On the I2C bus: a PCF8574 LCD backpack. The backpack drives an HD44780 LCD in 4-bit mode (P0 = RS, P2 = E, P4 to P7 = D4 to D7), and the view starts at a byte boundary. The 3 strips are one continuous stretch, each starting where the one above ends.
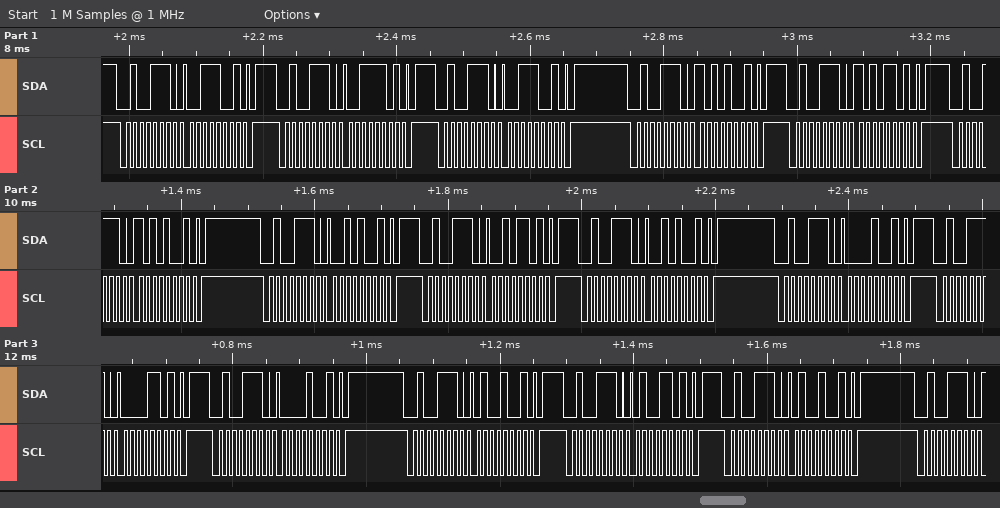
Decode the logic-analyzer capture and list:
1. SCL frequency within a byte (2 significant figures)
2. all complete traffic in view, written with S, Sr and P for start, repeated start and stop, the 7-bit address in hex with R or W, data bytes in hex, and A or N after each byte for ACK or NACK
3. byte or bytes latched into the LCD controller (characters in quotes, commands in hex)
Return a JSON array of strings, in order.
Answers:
["100 kHz", "S 27W A 39 A P S 27W A 3D A P S 27W A 39 A P S 27W A A9 A P S 27W A AD A P S 27W A A9 A P S 27W A 29 A P S 27W A 2D A P S 27W A 29 A P S 27W A 09 A P S 27W A 0D A P S 27W A 09 A P S 27W A 49 A P S 27W A 4D A P S 27W A 49 A P S 27W A", "':' ' '"]
